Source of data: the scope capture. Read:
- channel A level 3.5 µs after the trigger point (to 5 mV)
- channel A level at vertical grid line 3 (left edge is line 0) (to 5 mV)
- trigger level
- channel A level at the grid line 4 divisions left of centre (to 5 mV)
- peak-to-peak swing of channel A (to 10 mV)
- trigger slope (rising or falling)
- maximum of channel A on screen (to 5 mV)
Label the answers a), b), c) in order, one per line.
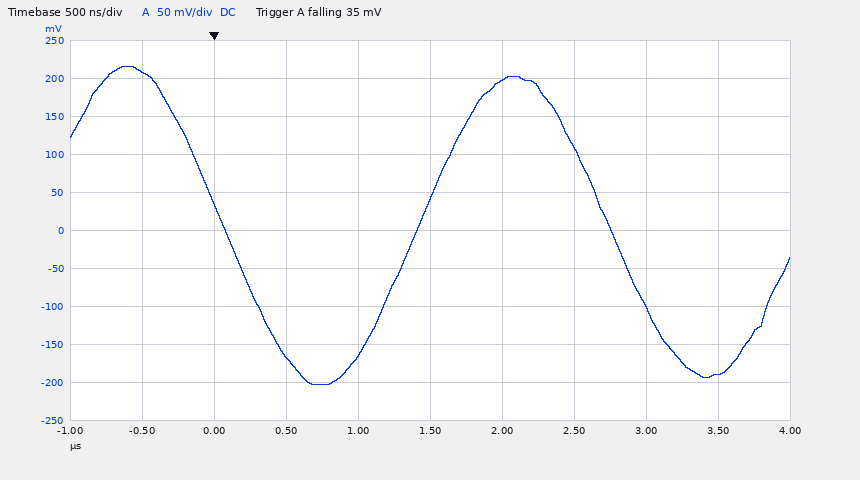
a) -190 mV
b) -165 mV
c) 35 mV
d) 210 mV
e) 420 mV
f) falling
g) 215 mV
